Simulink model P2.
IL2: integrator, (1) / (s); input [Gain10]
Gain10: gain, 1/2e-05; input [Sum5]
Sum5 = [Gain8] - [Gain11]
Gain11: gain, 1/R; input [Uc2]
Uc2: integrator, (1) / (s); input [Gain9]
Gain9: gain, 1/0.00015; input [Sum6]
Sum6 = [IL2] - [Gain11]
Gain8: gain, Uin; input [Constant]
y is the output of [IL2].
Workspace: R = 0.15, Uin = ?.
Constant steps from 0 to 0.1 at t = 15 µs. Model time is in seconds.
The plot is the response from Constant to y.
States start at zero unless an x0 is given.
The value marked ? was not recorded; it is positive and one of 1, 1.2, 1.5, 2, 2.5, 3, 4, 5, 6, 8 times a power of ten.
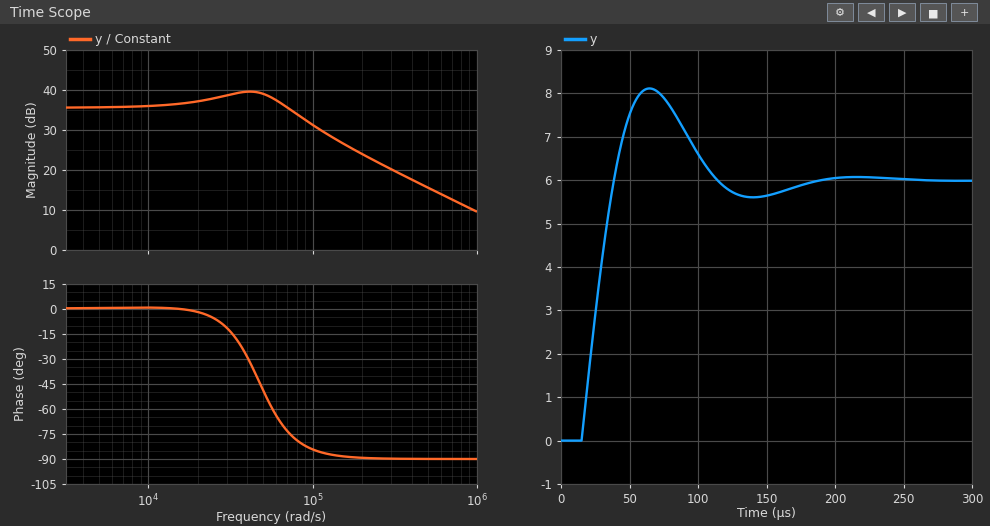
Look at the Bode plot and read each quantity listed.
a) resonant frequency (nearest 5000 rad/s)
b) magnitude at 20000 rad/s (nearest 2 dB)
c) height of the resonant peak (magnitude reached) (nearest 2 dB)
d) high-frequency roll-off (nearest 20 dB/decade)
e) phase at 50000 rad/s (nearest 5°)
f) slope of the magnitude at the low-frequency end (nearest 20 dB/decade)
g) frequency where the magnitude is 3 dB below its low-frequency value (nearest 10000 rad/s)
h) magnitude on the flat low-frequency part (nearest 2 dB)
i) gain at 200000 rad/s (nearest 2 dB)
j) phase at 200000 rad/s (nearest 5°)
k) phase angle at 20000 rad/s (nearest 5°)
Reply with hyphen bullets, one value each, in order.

- 40000 rad/s
- 38 dB
- 40 dB
- -20 dB/decade
- -50°
- 0 dB/decade
- 90000 rad/s
- 36 dB
- 24 dB
- -90°
- 0°
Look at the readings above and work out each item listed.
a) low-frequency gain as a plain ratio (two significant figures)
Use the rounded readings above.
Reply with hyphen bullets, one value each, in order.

- 63
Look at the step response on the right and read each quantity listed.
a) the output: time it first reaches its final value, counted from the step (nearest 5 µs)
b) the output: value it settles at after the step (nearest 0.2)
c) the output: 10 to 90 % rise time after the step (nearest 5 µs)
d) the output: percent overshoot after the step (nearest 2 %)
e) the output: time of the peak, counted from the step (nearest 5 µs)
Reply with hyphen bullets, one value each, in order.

- 25 µs
- 6.0
- 20 µs
- 36 %
- 50 µs
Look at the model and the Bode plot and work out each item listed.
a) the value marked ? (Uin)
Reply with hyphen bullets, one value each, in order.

- 60
